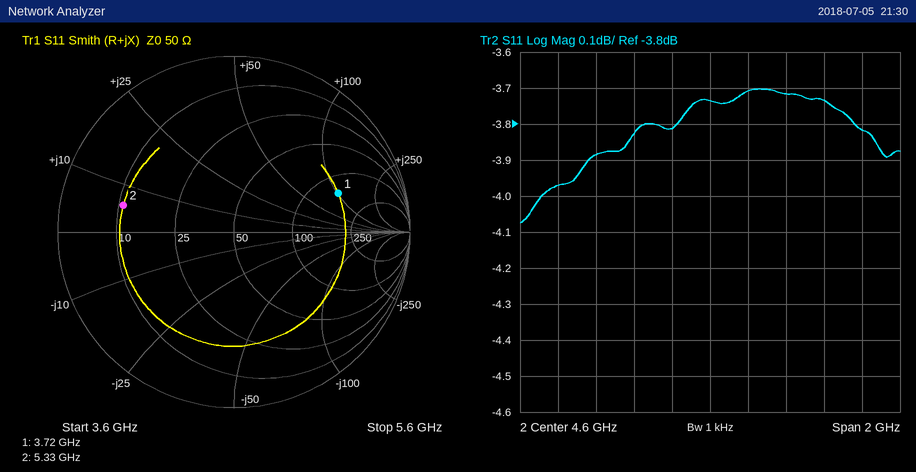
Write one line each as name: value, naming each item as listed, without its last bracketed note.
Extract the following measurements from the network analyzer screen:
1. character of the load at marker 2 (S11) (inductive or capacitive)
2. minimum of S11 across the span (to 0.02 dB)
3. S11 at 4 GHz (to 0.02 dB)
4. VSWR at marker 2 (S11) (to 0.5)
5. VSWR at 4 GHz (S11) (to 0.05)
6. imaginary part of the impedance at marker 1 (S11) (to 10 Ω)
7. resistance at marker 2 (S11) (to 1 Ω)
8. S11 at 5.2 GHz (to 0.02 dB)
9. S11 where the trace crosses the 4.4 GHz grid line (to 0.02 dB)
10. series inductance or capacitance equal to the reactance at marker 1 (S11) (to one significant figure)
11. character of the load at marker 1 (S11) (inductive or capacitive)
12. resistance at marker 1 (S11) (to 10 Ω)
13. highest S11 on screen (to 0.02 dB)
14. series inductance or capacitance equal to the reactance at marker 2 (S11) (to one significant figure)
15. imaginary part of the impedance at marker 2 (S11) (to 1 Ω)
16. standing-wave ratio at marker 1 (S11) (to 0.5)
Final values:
character of the load at marker 2 (S11): inductive
minimum of S11 across the span: -4.08 dB
S11 at 4 GHz: -3.88 dB
VSWR at marker 2 (S11): 4.5
VSWR at 4 GHz (S11): 4.55
imaginary part of the impedance at marker 1 (S11): +100 Ω
resistance at marker 2 (S11): 11 Ω
S11 at 5.2 GHz: -3.74 dB
S11 where the trace crosses the 4.4 GHz grid line: -3.82 dB
series inductance or capacitance equal to the reactance at marker 1 (S11): 4 nH
character of the load at marker 1 (S11): inductive
resistance at marker 1 (S11): 140 Ω
highest S11 on screen: -3.70 dB
series inductance or capacitance equal to the reactance at marker 2 (S11): 200 pH
imaginary part of the impedance at marker 2 (S11): +6 Ω
standing-wave ratio at marker 1 (S11): 4.5
